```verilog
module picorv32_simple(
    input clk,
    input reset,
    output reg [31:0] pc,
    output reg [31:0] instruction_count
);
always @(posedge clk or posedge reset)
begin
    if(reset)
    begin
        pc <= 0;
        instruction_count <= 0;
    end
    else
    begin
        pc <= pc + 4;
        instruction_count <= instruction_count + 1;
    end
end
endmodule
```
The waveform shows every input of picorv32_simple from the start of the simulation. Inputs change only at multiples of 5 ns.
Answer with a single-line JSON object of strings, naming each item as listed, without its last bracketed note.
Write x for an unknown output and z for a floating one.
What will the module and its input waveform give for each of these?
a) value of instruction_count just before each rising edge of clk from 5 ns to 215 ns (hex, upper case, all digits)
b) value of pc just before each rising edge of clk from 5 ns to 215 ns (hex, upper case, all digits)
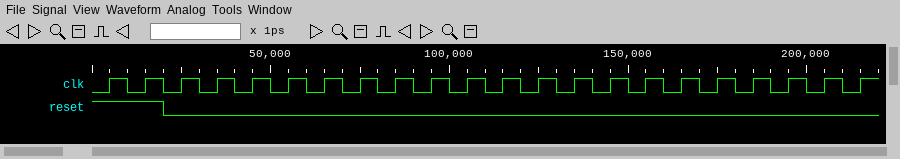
{"value of instruction_count just before each rising edge of clk from 5 ns to 215 ns": "00000000, 00000000, 00000000, 00000001, 00000002, 00000003, 00000004, 00000005, 00000006, 00000007, 00000008, 00000009, 0000000A, 0000000B, 0000000C, 0000000D, 0000000E, 0000000F, 00000010, 00000011, 00000012, 00000013", "value of pc just before each rising edge of clk from 5 ns to 215 ns": "00000000, 00000000, 00000000, 00000004, 00000008, 0000000C, 00000010, 00000014, 00000018, 0000001C, 00000020, 00000024, 00000028, 0000002C, 00000030, 00000034, 00000038, 0000003C, 00000040, 00000044, 00000048, 0000004C"}
